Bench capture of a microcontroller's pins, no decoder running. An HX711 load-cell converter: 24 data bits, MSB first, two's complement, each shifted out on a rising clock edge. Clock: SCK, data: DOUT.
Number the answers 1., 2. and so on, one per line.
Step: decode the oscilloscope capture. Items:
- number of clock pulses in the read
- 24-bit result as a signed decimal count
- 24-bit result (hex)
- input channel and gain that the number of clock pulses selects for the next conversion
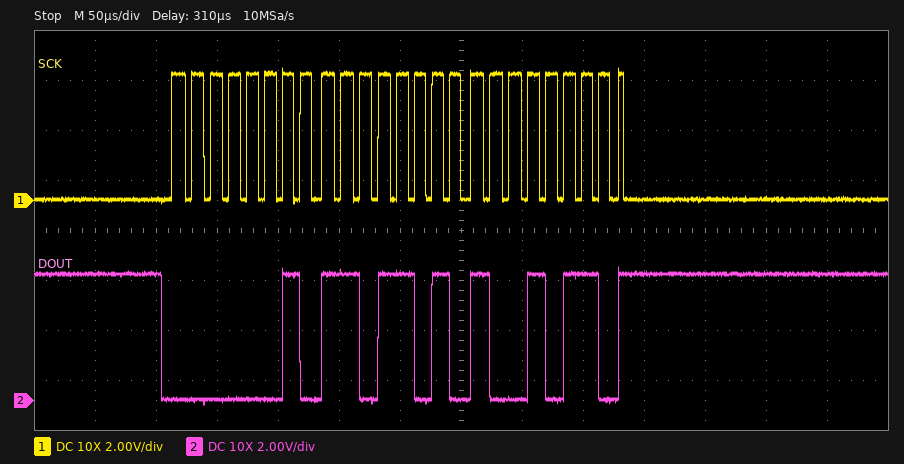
1. 25
2. 187030
3. 0x02DA96
4. channel A, gain 128
